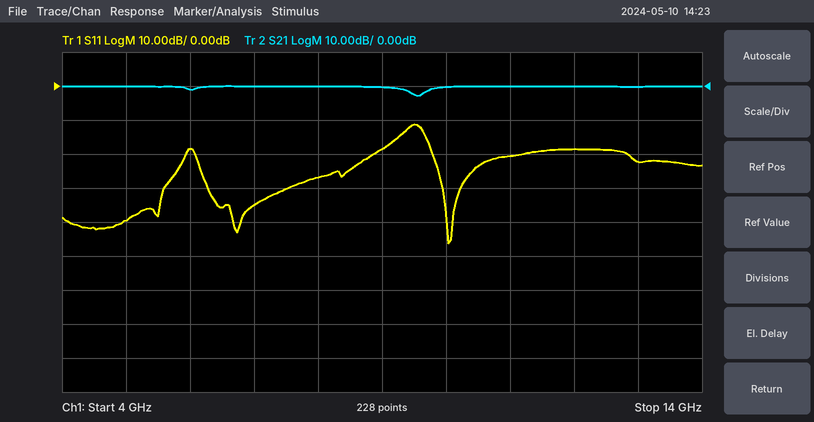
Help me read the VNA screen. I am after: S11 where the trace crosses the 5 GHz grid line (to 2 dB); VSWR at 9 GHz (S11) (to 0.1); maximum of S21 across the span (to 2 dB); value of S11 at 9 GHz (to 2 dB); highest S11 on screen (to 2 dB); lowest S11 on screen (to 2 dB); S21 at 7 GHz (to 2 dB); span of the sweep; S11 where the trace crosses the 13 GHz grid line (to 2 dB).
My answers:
-40 dB
1.3
0 dB
-18 dB
-12 dB
-46 dB
0 dB
10 GHz
-22 dB
